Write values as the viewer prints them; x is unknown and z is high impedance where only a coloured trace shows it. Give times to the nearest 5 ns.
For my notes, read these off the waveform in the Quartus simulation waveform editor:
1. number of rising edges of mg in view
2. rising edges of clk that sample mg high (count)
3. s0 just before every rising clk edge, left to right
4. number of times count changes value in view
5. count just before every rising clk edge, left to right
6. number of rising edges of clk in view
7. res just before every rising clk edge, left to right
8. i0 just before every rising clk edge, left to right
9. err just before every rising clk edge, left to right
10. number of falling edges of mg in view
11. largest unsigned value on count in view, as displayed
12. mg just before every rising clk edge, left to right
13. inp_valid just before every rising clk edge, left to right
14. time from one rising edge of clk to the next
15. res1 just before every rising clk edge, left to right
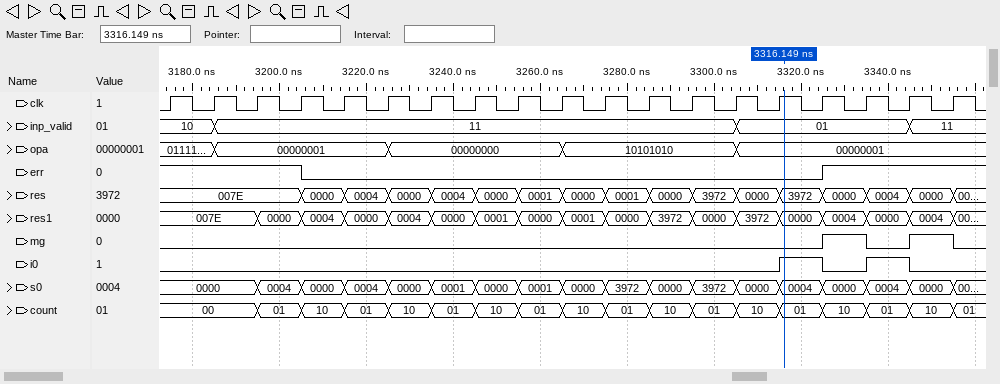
2
2
0000, 0000, 0000, 0004, 0000, 0004, 0000, 0001, 0000, 0001, 0000, 3972, 0000, 3972, 0000, 0004, 0000, 0004, 0000
17
00, 00, 00, 01, 10, 01, 10, 01, 10, 01, 10, 01, 10, 01, 10, 01, 10, 01, 10
19
007E, 007E, 007E, 007E, 0000, 0004, 0000, 0004, 0000, 0001, 0000, 0001, 0000, 3972, 0000, 3972, 0000, 0004, 0000
0 0 0 0 0 0 0 0 0 0 0 0 0 0 0 1 0 1 0
1 1 1 1 0 0 0 0 0 0 0 0 0 0 0 0 1 1 1
2
10
0 0 0 0 0 0 0 0 0 0 0 0 0 0 0 0 1 0 1
10, 10, 11, 11, 11, 11, 11, 11, 11, 11, 11, 11, 11, 11, 01, 01, 01, 01, 11
10 ns
007E, 007E, 007E, 0000, 0004, 0000, 0004, 0000, 0001, 0000, 0001, 0000, 3972, 0000, 3972, 0000, 0004, 0000, 0004
